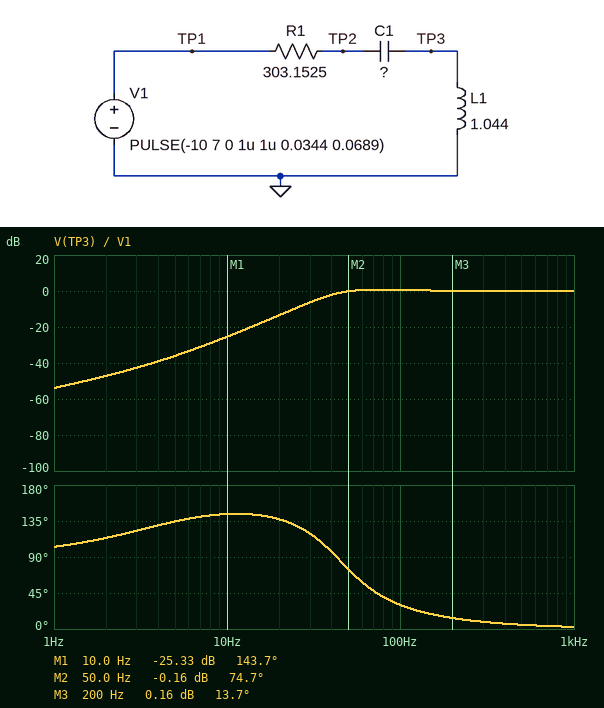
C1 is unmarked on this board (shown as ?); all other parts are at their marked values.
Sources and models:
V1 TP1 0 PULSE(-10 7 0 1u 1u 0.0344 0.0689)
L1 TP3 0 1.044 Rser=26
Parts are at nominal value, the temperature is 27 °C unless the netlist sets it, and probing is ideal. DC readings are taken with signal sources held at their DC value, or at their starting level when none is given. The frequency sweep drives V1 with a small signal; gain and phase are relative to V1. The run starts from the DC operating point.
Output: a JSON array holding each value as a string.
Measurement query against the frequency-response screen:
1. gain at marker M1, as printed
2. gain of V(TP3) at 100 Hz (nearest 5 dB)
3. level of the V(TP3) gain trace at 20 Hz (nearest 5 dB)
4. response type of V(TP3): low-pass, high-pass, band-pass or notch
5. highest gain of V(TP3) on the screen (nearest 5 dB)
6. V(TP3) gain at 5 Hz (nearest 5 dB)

["-25.33 dB", "0 dB", "-15 dB", "high-pass", "0 dB", "-35 dB"]
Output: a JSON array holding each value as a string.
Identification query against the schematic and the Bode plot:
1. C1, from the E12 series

["12 µF"]
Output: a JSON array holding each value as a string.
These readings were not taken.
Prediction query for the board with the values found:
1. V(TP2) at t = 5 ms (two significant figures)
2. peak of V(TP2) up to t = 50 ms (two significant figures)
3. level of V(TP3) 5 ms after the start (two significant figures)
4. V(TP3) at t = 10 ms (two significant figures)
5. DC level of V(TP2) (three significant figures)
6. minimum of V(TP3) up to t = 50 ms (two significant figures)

["-1.8 V", "8.1 V", "-1.0 V", "-3.9 V", "-10.0 V", "-17 V"]
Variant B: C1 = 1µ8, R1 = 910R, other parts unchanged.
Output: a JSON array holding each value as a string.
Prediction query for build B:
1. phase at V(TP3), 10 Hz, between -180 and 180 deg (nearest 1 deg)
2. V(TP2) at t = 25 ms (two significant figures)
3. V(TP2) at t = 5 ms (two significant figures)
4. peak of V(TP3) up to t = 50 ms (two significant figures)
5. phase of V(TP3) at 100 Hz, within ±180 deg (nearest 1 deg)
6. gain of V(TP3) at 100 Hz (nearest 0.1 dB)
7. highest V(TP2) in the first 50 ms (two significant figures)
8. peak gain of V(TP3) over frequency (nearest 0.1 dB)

["152 deg", "7.0 V", "6.3 V", "17 V", "101 deg", "-3.3 dB", "7.9 V", "0.3 dB"]
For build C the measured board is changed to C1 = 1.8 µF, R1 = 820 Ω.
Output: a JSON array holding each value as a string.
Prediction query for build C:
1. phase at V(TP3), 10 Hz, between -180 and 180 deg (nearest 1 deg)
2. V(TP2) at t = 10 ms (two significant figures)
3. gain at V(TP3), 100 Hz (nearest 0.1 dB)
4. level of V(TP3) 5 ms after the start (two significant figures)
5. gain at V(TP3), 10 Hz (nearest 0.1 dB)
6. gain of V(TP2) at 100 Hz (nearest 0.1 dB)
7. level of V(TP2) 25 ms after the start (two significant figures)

["153 deg", "7.1 V", "-2.5 dB", "-2.4 V", "-41.9 dB", "-11.6 dB", "7.0 V"]
